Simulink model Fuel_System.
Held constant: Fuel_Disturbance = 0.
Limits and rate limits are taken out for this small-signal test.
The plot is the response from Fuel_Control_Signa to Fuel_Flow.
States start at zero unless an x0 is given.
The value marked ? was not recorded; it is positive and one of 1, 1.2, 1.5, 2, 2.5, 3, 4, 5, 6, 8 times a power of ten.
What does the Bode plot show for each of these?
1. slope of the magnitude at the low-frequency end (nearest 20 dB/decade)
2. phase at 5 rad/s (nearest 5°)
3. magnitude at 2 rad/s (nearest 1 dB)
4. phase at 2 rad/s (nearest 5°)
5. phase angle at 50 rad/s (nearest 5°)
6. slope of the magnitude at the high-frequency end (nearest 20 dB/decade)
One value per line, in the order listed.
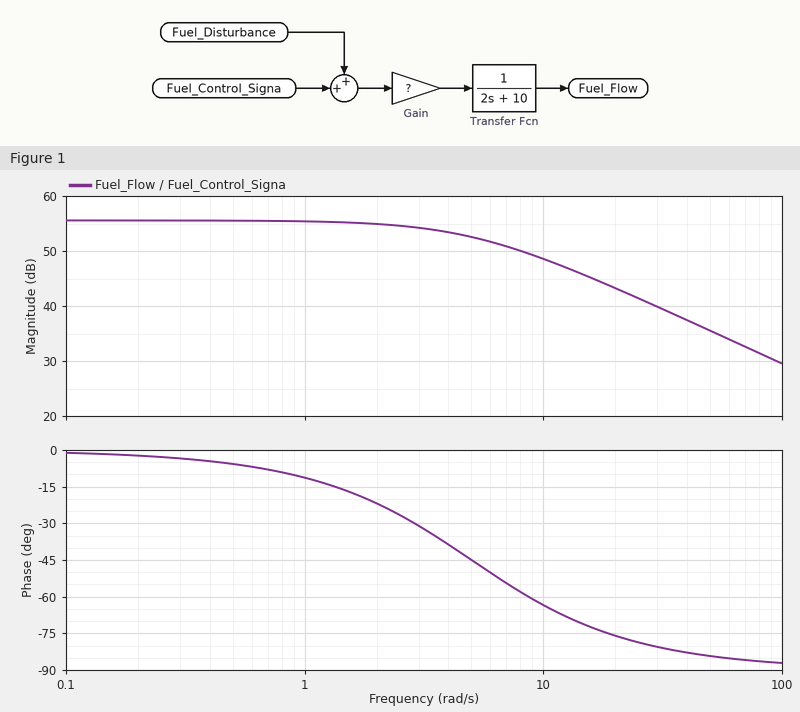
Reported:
0 dB/decade
-45°
55 dB
-20°
-85°
-20 dB/decade
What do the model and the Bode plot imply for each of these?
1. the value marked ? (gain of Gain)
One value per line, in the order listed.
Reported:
6000
